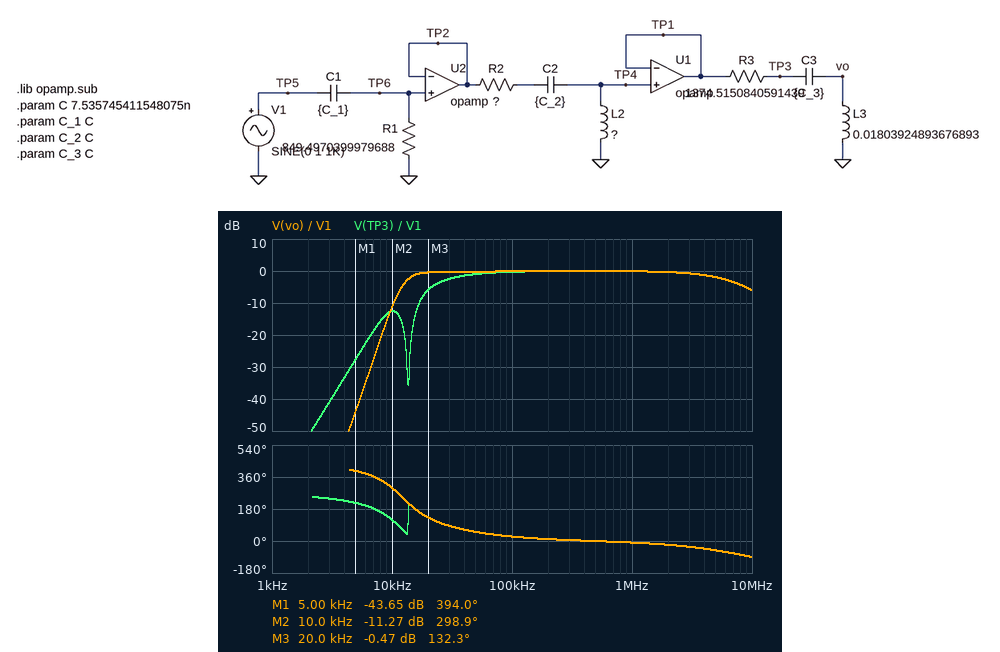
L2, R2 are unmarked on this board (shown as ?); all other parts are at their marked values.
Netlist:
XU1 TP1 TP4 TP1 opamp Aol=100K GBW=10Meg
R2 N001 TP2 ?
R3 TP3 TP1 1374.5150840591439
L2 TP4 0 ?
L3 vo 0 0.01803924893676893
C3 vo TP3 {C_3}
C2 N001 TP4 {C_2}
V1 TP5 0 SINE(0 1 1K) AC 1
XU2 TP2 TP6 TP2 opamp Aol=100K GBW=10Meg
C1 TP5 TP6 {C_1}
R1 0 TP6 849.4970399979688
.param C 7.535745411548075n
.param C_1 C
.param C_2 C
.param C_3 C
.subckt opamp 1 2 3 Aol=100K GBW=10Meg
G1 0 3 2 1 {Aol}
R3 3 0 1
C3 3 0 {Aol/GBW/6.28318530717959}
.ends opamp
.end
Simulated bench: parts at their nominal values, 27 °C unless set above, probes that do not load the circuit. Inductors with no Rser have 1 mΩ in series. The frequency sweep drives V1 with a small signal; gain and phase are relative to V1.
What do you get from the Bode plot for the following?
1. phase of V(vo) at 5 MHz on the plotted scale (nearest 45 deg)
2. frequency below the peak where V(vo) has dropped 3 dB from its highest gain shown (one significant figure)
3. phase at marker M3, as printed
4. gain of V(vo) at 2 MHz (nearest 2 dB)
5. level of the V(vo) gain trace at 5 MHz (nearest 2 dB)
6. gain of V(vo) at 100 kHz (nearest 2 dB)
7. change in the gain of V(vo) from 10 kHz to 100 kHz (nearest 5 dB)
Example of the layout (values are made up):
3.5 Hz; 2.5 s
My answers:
-45 deg; 10 kHz; 132.3 deg; 0 dB; -2 dB; 0 dB; 10 dB
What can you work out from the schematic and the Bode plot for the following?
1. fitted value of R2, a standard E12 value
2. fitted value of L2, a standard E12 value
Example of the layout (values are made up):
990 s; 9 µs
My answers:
1.5 kΩ; 27 mH
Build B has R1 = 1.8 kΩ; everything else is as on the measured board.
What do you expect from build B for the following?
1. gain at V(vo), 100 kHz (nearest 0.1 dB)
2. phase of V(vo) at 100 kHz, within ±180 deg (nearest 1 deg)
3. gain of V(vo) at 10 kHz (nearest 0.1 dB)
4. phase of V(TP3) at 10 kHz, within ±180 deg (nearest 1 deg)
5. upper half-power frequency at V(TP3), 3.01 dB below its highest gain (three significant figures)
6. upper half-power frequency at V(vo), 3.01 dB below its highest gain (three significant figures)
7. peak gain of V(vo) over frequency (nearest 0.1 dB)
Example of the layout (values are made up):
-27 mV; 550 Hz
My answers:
0.1 dB; 18 deg; -6.5 dB; 100 deg; 6.45 MHz; 2.36 MHz; 2.5 dB
